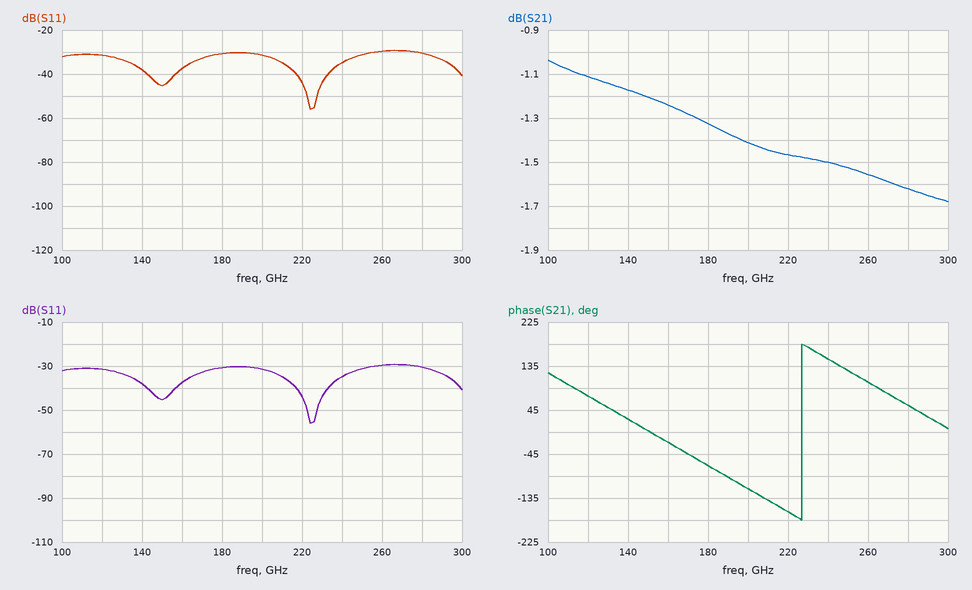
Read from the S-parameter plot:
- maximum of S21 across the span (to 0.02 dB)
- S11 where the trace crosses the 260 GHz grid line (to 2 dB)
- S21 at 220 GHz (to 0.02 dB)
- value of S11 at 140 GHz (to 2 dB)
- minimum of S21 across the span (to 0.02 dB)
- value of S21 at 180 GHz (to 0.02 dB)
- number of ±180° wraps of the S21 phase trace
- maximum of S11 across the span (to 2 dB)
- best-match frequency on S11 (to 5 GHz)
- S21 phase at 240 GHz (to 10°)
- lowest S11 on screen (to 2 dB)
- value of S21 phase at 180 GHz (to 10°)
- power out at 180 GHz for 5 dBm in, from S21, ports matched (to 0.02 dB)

-1.04 dB
-30 dB
-1.46 dB
-38 dB
-1.68 dB
-1.32 dB
1
-30 dB
225 GHz
150°
-56 dB
-70°
3.68 dBm
